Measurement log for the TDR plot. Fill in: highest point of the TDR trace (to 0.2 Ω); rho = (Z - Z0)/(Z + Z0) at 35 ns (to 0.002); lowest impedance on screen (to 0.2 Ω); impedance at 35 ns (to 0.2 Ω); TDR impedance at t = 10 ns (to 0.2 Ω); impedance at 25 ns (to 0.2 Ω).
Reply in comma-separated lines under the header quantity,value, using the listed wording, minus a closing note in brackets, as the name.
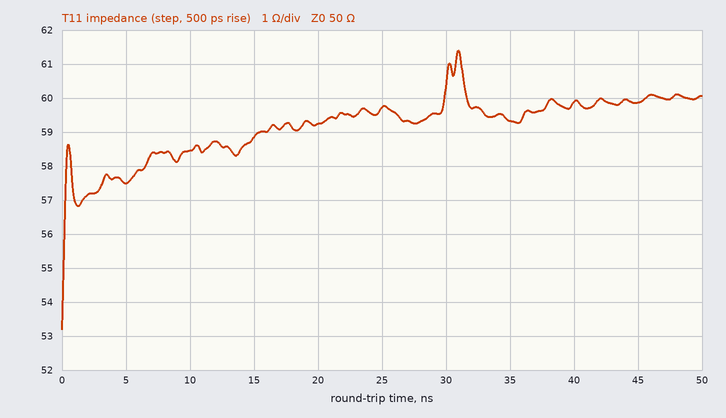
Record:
quantity,value
highest point of the TDR trace,61.4 Ω
rho = (Z - Z0)/(Z + Z0) at 35 ns,+0.086
lowest impedance on screen,53.2 Ω
impedance at 35 ns,59.4 Ω
TDR impedance at t = 10 ns,58.4 Ω
impedance at 25 ns,59.8 Ω
